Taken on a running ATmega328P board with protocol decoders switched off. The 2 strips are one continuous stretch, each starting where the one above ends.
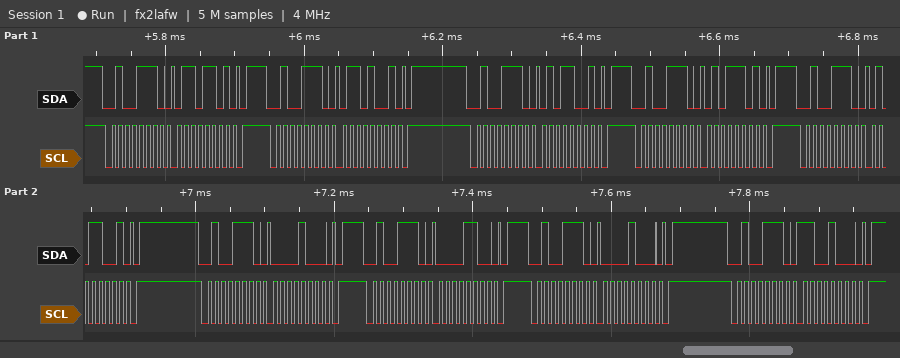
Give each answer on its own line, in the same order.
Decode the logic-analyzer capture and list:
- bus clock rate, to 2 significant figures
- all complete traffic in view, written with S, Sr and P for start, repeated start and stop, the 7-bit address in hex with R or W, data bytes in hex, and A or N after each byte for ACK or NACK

100 kHz
S 27W A 6D A P S 27W A 69 A P S 27W A 59 A P S 27W A 5D A P S 27W A 59 A P S 27W A 08 A P S 27W A 0C A P S 27W A 08 A P S 27W A C8 A P
